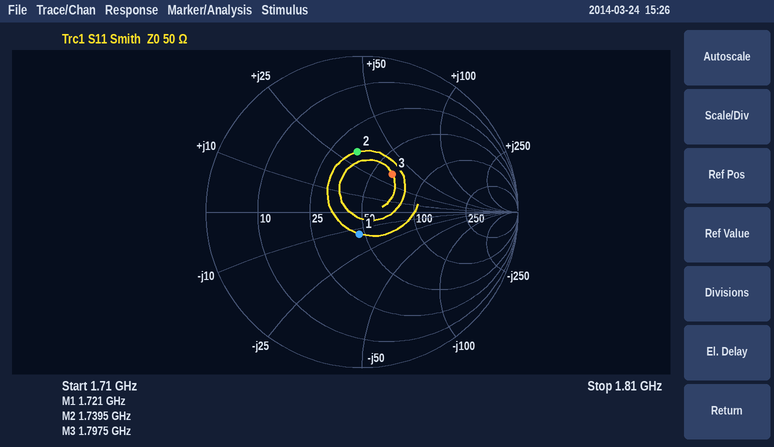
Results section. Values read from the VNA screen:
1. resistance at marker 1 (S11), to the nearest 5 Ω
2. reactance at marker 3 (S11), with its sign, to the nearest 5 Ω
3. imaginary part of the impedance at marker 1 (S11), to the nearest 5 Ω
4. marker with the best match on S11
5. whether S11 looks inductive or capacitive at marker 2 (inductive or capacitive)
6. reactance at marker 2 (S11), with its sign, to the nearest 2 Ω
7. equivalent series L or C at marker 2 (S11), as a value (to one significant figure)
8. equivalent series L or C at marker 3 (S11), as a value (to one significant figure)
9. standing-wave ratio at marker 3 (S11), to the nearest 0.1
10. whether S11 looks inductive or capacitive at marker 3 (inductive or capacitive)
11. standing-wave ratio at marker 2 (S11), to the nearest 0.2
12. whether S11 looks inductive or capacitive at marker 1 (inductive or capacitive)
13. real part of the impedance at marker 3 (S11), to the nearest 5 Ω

45 Ω
+35 Ω
-15 Ω
marker 1
inductive
+32 Ω
3 nH
3 nH
1.9
inductive
2.2
capacitive
65 Ω
